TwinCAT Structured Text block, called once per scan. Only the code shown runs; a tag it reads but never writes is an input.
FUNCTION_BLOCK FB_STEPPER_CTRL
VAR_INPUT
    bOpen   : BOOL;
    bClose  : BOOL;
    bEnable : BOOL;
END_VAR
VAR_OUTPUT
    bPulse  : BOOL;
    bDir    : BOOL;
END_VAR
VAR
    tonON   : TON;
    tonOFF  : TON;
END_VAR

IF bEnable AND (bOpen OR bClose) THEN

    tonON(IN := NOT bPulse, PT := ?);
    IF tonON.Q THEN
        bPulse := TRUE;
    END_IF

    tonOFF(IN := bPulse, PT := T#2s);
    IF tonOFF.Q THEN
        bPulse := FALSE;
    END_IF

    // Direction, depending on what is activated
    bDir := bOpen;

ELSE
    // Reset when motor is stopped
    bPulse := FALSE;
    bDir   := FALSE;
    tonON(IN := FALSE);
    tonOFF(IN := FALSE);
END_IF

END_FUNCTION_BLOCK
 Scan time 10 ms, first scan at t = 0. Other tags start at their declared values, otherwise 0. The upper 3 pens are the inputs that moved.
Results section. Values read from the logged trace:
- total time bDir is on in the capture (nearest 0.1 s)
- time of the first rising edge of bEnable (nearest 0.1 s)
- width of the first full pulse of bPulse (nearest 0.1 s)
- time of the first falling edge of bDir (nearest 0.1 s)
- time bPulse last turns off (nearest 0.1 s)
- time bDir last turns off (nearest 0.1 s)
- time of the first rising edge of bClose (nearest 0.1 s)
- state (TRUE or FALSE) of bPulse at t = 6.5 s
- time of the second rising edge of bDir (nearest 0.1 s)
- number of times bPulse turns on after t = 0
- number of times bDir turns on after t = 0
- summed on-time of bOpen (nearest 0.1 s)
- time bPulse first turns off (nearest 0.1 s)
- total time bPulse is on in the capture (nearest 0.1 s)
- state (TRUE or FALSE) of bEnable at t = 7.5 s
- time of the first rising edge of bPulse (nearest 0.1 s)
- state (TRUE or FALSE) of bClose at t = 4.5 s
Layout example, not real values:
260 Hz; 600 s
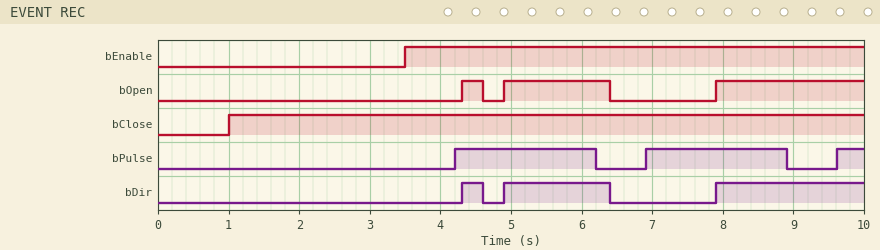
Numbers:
3.9 s; 3.5 s; 2.0 s; 4.6 s; 8.9 s; 6.4 s; 1.0 s; FALSE; 4.9 s; 3; 3; 3.9 s; 6.2 s; 4.4 s; TRUE; 4.2 s; TRUE
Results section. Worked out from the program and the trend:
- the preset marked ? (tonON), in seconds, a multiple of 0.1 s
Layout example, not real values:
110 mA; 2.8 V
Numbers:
0.7 s
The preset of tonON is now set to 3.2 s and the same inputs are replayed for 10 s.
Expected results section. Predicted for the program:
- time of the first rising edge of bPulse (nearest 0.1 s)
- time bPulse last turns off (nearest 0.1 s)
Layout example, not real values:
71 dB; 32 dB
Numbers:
6.7 s; 8.7 s
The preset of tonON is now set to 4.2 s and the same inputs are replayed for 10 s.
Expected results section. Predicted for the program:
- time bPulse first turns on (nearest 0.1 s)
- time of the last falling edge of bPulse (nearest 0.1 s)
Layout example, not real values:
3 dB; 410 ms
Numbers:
7.7 s; 9.7 s
